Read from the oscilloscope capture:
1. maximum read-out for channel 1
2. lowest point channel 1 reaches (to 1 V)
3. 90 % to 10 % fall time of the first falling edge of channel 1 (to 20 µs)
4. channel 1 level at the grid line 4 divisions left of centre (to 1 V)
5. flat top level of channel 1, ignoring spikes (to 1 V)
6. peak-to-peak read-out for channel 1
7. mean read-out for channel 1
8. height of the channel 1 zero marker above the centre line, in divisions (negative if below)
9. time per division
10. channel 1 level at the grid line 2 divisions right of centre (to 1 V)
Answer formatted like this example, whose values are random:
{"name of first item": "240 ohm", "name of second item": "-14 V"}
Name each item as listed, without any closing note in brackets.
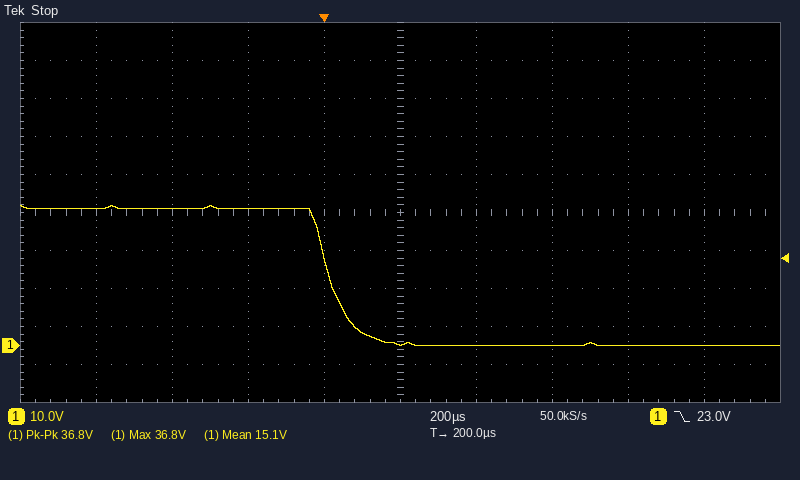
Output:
{"maximum read-out for channel 1": "36.8 V", "lowest point channel 1 reaches": "0 V", "90 % to 10 % fall time of the first falling edge of channel 1": "120 µs", "channel 1 level at the grid line 4 divisions left of centre": "36 V", "flat top level of channel 1, ignoring spikes": "36 V", "peak-to-peak read-out for channel 1": "36.8 V", "mean read-out for channel 1": "15.1 V", "height of the channel 1 zero marker above the centre line, in divisions": "-3.5 div", "time per division": "200 µs", "channel 1 level at the grid line 2 divisions right of centre": "0 V"}
